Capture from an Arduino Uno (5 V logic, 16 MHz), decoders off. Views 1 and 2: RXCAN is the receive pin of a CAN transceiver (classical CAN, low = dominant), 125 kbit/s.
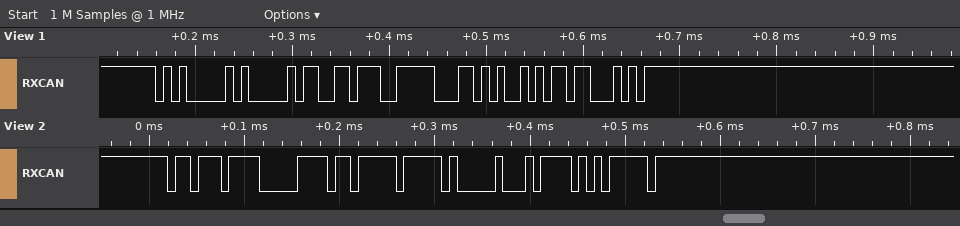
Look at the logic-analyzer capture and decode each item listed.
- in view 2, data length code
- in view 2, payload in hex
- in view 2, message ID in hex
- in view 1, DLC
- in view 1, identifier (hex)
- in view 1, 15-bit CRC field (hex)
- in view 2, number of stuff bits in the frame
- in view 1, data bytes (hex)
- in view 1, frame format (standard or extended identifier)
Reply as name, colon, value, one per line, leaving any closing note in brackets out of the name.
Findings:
in view 2, data length code: 3
in view 2, payload in hex: B7 FF 00
in view 2, message ID in hex: 0x6EF
in view 1, DLC: 3
in view 1, identifier: 0x502
in view 1, 15-bit CRC field: 0x2B62
in view 2, number of stuff bits in the frame: 4
in view 1, data bytes: 37 3E 6A
in view 1, frame format: standard
